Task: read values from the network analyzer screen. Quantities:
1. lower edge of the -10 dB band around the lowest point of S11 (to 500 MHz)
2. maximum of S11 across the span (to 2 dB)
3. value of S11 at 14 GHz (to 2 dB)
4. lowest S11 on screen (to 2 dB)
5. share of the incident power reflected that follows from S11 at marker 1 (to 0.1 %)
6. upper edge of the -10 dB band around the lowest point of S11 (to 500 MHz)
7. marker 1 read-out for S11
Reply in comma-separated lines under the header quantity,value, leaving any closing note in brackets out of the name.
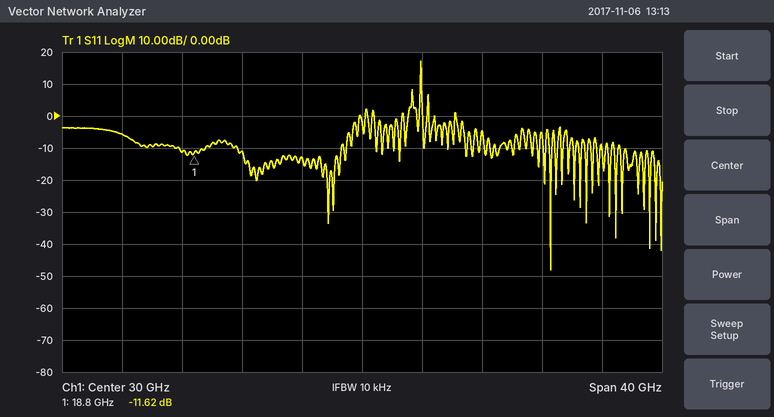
quantity,value
lower edge of the -10 dB band around the lowest point of S11,42.5 GHz
maximum of S11 across the span,18 dB
value of S11 at 14 GHz,-6 dB
lowest S11 on screen,-48 dB
share of the incident power reflected that follows from S11 at marker 1,6.9 %
upper edge of the -10 dB band around the lowest point of S11,42.5 GHz
marker 1 read-out for S11,-11.62 dB
